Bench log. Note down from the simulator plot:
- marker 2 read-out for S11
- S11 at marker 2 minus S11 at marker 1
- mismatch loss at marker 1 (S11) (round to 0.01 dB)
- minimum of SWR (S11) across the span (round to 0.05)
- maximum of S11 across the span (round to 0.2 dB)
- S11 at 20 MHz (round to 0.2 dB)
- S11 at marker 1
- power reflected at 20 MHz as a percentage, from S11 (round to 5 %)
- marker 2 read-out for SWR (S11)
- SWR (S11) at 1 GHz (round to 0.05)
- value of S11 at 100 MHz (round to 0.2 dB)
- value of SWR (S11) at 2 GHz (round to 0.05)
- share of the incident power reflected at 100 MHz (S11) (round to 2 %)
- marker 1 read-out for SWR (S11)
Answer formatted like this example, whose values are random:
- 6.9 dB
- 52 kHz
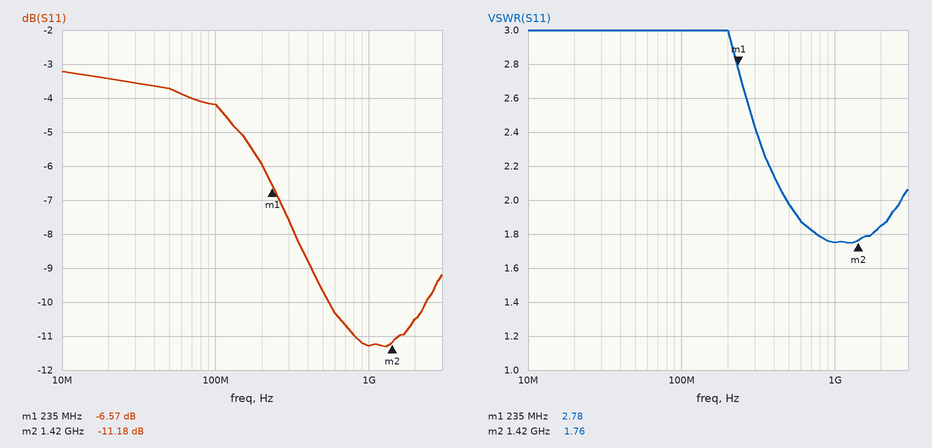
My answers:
- -11.18 dB
- -4.61 dB
- 1.08 dB
- 1.75
- -3.2 dB
- -3.4 dB
- -6.57 dB
- 45 %
- 1.76
- 1.75
- -4.2 dB
- 1.85
- 38 %
- 2.78
